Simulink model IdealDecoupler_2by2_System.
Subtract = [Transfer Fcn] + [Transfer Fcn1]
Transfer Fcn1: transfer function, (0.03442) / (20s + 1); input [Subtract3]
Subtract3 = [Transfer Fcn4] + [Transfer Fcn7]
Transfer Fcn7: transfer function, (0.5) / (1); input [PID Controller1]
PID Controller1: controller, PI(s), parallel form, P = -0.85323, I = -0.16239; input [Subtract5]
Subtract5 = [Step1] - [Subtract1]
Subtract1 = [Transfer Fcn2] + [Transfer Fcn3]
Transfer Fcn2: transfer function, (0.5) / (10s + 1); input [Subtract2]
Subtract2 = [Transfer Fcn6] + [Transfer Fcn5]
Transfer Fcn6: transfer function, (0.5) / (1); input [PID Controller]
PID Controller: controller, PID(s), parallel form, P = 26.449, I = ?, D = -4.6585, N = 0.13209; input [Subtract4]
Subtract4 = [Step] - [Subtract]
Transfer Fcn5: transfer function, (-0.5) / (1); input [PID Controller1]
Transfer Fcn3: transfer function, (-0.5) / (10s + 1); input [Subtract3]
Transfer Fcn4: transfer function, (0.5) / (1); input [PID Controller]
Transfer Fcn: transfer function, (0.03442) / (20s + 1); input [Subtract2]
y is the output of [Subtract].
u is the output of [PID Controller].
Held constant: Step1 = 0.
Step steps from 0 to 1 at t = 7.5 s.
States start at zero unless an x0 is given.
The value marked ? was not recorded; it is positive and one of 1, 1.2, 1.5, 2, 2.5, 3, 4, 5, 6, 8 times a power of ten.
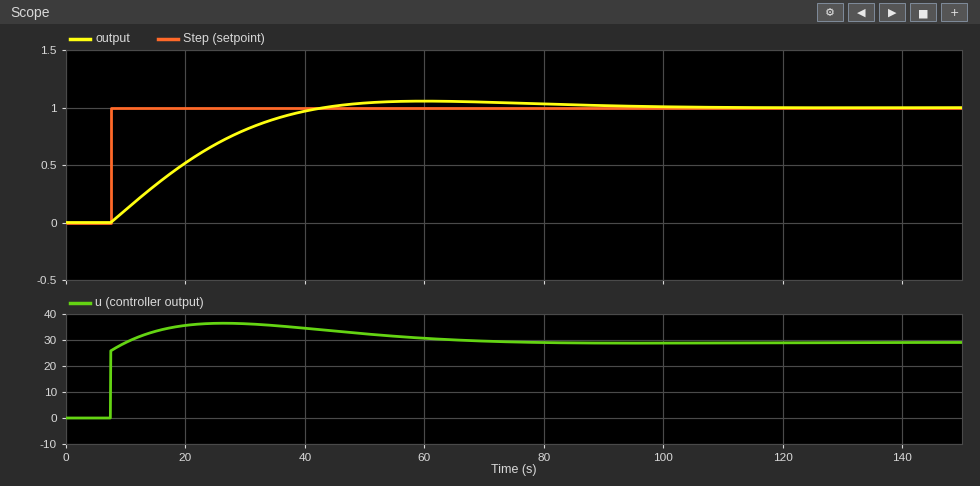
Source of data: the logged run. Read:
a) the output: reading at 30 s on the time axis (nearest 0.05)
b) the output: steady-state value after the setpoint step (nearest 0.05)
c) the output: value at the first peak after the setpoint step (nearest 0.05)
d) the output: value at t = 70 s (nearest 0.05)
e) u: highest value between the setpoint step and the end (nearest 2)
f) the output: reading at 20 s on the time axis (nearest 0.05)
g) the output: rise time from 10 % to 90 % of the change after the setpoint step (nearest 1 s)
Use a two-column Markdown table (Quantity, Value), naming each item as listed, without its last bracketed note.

| Quantity | Value |
|---|---|
| the output: reading at 30 s on the time axis | 0.80 |
| the output: steady-state value after the setpoint step | 1.00 |
| the output: value at the first peak after the setpoint step | 1.05 |
| the output: value at t = 70 s | 1.05 |
| u: highest value between the setpoint step and the end | 36 |
| the output: reading at 20 s on the time axis | 0.50 |
| the output: rise time from 10 % to 90 % of the change after the setpoint step | 25 s |
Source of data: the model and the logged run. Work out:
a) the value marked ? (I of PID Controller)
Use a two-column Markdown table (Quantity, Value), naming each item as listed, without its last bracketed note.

| Quantity | Value |
|---|---|
| the value marked ? | 2.5 |
